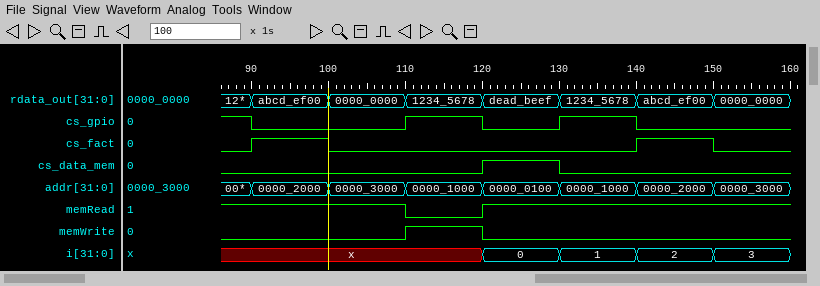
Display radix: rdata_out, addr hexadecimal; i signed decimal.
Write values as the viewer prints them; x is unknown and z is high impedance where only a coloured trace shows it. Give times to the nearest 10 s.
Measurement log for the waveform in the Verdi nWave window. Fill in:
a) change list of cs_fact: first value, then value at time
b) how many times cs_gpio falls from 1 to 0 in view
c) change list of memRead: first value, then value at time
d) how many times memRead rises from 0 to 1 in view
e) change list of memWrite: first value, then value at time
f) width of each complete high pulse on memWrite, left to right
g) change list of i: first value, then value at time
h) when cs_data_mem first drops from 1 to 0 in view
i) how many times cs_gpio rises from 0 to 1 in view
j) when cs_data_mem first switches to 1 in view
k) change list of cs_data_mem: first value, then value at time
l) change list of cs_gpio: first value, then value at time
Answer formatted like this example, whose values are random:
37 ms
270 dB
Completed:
0, 1 at 90 s, 0 at 100 s, 1 at 140 s, 0 at 150 s
3
1, 0 at 110 s, 1 at 120 s
1
0, 1 at 110 s, 0 at 120 s
10 s
x, 0 at 120 s, 1 at 130 s, 2 at 140 s, 3 at 150 s
130 s
2
120 s
0, 1 at 120 s, 0 at 130 s
1, 0 at 90 s, 1 at 110 s, 0 at 120 s, 1 at 130 s, 0 at 140 s
